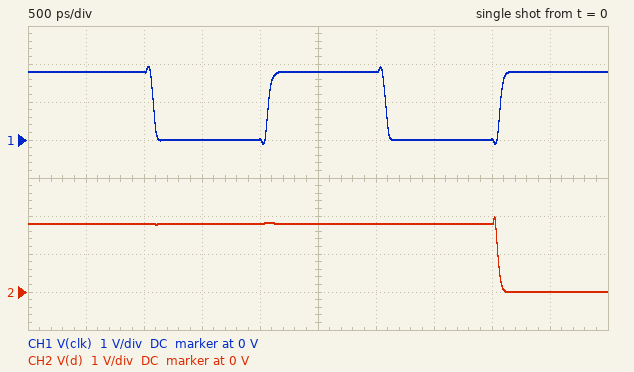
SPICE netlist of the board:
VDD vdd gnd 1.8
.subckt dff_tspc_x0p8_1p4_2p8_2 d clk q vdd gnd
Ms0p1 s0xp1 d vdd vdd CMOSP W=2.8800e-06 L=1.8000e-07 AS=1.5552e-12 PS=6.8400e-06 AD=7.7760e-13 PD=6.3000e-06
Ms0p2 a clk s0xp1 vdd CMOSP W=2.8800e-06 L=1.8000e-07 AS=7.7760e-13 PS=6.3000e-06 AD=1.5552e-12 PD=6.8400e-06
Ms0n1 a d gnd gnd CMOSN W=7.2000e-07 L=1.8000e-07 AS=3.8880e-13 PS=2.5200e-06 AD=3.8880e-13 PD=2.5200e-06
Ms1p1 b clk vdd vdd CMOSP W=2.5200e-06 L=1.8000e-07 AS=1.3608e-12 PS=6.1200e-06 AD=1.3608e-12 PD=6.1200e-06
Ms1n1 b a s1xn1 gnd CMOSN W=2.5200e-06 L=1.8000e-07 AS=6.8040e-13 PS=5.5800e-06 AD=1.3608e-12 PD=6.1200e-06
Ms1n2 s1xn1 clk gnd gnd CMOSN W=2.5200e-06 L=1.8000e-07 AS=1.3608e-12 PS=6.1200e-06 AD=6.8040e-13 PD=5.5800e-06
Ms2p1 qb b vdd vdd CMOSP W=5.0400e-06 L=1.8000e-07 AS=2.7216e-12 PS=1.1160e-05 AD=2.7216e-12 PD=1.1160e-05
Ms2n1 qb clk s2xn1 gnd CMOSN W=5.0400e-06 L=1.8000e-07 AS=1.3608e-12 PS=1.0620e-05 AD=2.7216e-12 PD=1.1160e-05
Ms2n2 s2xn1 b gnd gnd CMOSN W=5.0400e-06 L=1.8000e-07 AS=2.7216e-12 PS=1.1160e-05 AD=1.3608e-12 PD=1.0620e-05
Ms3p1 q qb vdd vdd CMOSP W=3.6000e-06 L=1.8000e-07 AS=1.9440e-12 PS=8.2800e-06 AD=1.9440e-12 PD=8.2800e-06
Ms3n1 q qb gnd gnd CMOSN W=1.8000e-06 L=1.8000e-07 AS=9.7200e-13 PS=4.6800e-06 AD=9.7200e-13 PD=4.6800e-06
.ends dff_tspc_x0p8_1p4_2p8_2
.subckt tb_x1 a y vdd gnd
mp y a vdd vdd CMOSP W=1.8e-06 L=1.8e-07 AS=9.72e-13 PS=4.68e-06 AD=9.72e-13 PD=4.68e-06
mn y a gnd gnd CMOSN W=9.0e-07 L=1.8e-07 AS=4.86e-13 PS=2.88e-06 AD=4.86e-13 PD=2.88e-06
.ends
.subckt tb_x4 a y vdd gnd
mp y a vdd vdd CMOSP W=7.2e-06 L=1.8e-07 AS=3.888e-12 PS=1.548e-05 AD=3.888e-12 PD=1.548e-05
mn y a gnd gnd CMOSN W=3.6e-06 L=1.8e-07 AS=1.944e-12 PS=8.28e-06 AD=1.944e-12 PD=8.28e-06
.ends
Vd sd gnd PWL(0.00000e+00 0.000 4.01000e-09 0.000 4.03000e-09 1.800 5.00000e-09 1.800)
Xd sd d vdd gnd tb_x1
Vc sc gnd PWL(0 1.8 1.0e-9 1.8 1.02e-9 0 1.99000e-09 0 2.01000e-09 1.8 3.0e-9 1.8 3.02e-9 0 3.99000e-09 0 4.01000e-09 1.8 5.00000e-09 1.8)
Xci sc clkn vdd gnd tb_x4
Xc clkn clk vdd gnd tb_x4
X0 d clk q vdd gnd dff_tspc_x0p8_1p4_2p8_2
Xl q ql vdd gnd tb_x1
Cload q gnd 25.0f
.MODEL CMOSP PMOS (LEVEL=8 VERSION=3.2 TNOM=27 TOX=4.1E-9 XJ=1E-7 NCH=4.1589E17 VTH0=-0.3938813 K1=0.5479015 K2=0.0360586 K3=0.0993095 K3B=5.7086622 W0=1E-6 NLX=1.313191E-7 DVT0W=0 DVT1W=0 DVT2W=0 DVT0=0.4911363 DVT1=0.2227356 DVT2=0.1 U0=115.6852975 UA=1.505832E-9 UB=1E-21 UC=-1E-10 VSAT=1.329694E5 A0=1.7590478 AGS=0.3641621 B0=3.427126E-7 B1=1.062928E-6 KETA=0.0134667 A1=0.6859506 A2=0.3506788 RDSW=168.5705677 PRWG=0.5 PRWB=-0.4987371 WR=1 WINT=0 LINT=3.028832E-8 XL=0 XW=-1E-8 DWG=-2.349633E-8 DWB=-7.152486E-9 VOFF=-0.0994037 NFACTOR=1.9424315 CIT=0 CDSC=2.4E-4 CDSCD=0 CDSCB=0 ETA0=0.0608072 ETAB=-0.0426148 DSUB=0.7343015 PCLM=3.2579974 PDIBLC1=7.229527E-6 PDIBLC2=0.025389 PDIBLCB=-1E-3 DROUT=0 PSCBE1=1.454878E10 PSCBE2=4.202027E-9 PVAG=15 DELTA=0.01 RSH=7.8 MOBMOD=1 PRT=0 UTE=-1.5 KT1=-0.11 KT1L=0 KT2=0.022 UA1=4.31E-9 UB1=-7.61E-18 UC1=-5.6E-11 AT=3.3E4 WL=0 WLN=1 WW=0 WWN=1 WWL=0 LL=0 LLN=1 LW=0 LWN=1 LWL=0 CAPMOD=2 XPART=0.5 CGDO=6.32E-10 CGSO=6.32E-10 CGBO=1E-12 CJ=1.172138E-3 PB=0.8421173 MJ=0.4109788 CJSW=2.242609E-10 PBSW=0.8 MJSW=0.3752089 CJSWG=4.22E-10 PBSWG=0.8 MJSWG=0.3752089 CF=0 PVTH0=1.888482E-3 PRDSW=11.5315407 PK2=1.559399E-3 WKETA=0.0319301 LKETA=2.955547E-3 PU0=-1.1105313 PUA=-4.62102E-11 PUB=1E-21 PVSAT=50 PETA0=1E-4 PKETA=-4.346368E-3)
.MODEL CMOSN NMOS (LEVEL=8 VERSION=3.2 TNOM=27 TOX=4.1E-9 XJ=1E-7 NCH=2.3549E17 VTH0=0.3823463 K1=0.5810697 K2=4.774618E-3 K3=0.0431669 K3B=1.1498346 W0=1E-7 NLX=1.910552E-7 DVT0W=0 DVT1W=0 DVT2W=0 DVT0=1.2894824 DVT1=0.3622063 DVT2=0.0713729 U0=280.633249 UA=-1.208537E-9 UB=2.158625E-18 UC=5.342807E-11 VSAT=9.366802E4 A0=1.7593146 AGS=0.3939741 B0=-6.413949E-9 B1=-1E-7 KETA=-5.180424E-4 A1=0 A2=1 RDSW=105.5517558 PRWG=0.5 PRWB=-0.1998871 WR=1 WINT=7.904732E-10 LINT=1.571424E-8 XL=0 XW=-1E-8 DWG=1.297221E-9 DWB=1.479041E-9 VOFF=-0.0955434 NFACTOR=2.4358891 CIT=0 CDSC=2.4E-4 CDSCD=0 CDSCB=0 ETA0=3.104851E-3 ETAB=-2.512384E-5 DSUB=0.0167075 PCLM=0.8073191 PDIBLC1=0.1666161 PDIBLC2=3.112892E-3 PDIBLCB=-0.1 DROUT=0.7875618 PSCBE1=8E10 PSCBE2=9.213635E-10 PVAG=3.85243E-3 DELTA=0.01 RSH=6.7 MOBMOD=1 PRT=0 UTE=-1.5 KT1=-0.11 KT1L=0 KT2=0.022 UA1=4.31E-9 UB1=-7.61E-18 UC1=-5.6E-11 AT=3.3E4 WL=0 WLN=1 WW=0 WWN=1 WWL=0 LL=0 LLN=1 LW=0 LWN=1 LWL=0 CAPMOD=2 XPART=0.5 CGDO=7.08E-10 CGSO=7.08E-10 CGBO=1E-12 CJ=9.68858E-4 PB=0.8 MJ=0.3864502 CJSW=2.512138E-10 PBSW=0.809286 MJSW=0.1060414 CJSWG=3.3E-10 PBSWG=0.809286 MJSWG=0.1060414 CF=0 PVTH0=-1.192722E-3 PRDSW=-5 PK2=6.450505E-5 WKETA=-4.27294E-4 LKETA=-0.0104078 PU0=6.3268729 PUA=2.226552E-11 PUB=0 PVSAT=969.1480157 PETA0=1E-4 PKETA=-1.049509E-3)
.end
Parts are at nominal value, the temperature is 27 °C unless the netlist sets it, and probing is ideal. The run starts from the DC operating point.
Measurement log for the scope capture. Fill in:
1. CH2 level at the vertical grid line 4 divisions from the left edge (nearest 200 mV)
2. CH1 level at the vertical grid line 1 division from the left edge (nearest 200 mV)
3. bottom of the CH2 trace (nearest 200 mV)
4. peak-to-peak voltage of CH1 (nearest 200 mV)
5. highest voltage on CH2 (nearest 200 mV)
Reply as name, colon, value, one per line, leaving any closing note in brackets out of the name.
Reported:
CH2 level at the vertical grid line 4 divisions from the left edge: 1.8 V
CH1 level at the vertical grid line 1 division from the left edge: 1.8 V
bottom of the CH2 trace: 0 V
peak-to-peak voltage of CH1: 2.0 V
highest voltage on CH2: 2.0 V
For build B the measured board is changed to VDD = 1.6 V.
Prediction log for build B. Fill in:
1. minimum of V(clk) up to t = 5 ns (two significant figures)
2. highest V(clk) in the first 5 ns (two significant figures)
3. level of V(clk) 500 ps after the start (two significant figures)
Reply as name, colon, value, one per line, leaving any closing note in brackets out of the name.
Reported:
minimum of V(clk) up to t = 5 ns: -120 mV
highest V(clk) in the first 5 ns: 1.7 V
level of V(clk) 500 ps after the start: 1.6 V
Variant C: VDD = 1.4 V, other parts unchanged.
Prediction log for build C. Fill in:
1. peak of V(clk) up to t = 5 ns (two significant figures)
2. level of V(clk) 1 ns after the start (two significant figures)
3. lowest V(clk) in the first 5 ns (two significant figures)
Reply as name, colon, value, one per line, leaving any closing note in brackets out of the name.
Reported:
peak of V(clk) up to t = 5 ns: 1.5 V
level of V(clk) 1 ns after the start: 1.4 V
lowest V(clk) in the first 5 ns: -140 mV
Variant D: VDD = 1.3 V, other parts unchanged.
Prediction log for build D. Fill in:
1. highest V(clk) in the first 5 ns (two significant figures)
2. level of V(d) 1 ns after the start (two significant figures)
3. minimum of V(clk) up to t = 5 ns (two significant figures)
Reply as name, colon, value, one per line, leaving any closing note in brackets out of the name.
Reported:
highest V(clk) in the first 5 ns: 1.4 V
level of V(d) 1 ns after the start: 1.3 V
minimum of V(clk) up to t = 5 ns: -150 mV
